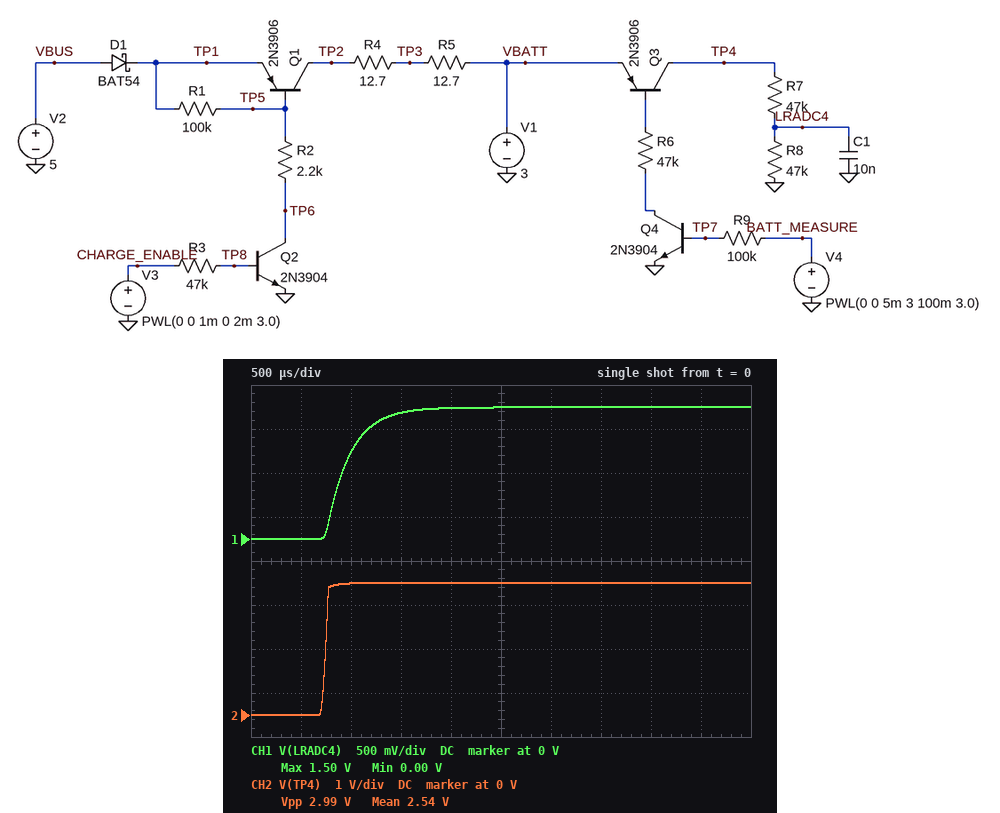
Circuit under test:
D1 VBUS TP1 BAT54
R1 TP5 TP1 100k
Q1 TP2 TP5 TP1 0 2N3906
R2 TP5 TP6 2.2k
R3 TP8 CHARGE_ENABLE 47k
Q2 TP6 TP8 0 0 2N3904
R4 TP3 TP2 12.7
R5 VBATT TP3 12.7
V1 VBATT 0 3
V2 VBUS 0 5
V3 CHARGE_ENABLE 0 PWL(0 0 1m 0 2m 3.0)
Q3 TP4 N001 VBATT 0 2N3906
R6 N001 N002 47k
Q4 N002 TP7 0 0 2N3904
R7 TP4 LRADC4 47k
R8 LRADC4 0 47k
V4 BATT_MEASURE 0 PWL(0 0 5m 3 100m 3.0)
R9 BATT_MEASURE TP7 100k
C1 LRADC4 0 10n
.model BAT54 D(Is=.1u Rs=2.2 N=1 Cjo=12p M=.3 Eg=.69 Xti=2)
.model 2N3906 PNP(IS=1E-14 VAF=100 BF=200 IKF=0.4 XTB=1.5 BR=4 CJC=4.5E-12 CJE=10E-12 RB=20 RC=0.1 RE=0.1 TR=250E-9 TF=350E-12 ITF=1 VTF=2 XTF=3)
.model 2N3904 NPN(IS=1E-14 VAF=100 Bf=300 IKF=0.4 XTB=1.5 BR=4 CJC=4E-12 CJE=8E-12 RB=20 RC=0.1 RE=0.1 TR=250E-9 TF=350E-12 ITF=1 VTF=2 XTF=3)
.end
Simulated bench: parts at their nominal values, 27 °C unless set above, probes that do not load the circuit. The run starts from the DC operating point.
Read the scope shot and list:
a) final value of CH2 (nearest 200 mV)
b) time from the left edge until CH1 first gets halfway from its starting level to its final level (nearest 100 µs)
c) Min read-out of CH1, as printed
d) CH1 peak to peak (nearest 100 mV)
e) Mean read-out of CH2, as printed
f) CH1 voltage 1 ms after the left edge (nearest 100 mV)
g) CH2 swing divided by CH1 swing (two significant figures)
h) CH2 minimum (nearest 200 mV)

3.0 V
900 µs
0.00 V
1.5 V
2.54 V
1.0 V
2.0
0 V
